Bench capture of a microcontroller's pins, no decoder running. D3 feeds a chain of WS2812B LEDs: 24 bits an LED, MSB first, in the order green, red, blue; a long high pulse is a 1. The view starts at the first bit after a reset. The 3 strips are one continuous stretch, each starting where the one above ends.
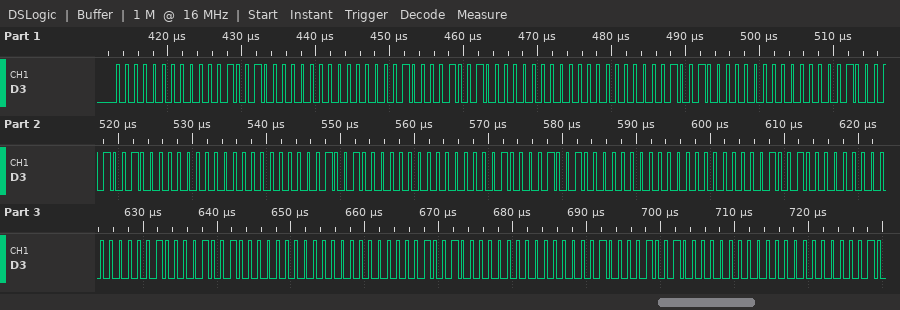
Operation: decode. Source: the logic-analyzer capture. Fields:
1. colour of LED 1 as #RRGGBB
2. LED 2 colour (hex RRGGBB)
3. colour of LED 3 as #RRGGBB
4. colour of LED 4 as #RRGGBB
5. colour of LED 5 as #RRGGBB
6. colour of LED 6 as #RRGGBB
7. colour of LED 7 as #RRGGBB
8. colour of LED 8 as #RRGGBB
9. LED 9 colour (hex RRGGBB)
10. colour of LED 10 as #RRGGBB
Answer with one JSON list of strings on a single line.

["#090000", "#090100", "#090000", "#090100", "#090000", "#090100", "#090000", "#090100", "#090000", "#090100"]
